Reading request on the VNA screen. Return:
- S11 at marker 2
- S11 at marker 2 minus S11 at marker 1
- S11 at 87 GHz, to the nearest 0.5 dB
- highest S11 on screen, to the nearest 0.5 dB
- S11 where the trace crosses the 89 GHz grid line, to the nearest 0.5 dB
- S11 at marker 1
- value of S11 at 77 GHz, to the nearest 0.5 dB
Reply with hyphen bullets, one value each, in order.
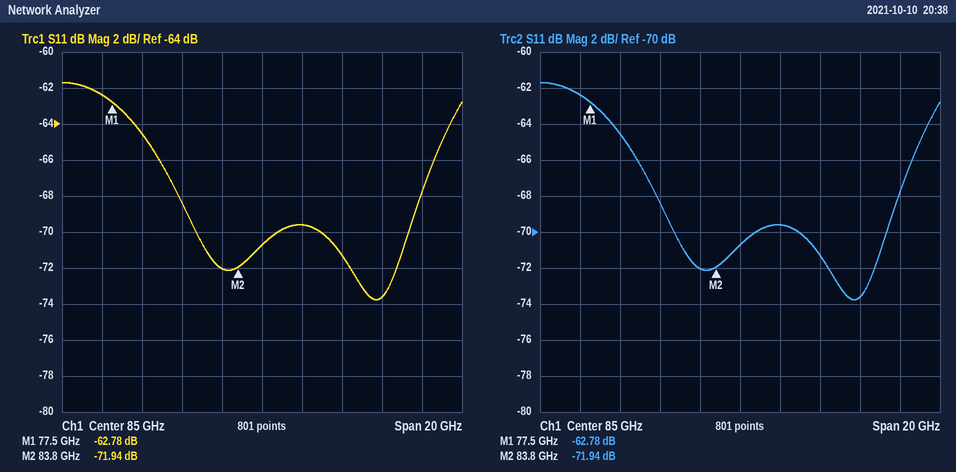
- -71.94 dB
- -9.16 dB
- -69.5 dB
- -61.5 dB
- -71.5 dB
- -62.78 dB
- -62.5 dB
